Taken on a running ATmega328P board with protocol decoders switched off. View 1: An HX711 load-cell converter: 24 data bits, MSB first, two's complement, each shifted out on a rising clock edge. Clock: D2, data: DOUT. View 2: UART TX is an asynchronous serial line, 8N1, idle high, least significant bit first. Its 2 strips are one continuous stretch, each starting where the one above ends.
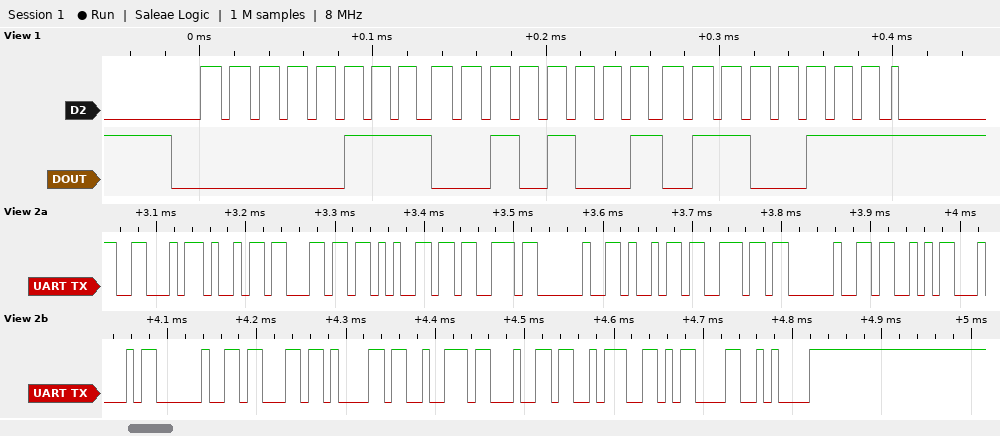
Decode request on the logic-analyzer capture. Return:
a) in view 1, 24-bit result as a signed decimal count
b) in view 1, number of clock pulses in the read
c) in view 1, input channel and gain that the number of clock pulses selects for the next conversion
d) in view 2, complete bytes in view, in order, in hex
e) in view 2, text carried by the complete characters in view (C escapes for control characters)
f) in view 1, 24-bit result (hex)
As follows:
469351
25
channel A, gain 128
46 69 6C 65 73 20 69 6E 20 53 44 20 63 61 72 64 3A 0D 0A
"Files in SD card:\r\n"
0x072967
